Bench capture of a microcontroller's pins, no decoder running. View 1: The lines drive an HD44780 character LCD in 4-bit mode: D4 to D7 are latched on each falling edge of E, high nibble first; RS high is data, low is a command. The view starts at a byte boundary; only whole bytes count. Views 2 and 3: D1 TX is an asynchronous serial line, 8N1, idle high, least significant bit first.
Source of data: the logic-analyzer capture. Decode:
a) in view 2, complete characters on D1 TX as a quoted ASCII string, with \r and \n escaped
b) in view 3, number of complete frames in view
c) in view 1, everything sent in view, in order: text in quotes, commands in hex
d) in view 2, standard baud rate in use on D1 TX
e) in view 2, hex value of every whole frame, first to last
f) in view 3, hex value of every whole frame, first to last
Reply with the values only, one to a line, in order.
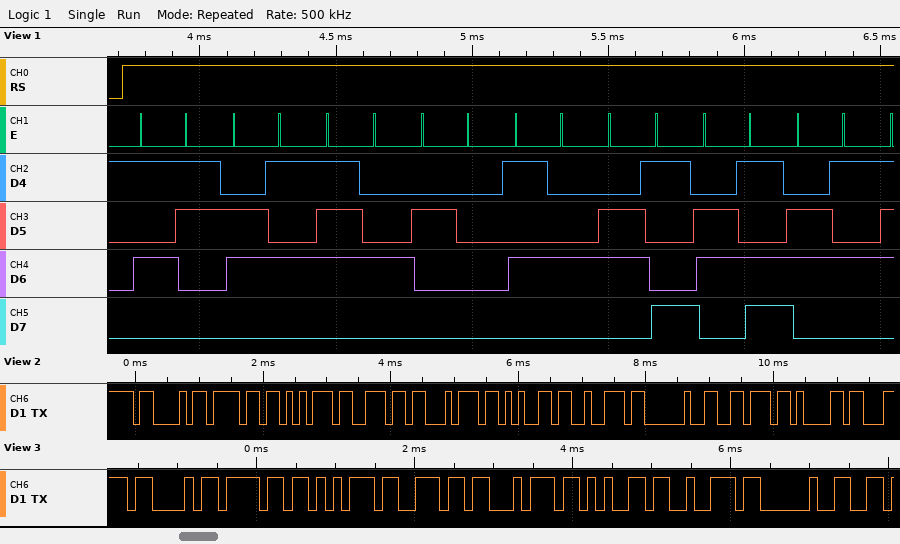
"Counter va"
8
"Set Time"
9600 baud
43 6F 75 6E 74 65 72 20 76 61
43 6F 75 6E 74 65 72 20
